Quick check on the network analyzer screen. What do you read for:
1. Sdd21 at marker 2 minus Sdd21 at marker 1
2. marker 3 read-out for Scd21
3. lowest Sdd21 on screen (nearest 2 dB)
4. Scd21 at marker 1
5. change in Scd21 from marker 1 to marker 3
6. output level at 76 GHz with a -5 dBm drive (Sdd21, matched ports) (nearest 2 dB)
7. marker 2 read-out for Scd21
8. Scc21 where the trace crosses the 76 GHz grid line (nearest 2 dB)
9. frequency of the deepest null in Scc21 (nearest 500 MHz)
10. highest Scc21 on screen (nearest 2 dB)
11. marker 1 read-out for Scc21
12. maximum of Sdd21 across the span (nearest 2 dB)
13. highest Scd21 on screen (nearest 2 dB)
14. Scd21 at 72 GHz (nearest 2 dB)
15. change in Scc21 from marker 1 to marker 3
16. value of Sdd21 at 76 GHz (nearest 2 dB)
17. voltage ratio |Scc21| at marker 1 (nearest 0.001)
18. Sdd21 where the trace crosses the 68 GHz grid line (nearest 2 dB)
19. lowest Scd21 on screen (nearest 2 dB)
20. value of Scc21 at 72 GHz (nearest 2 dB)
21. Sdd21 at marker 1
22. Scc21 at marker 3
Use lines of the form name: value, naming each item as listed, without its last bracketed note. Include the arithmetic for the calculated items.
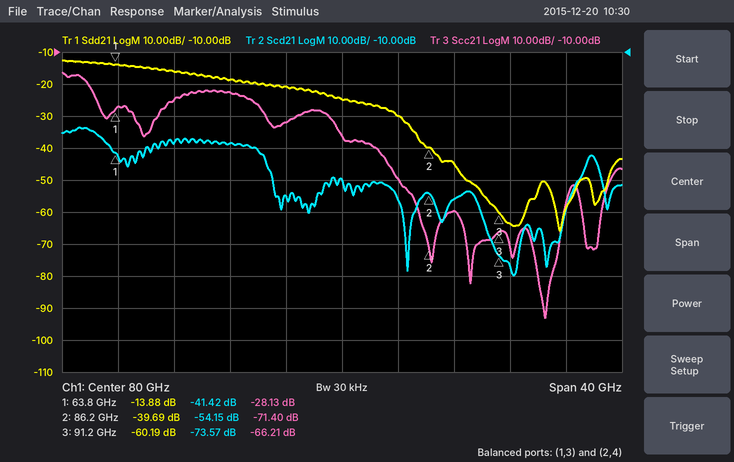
Sdd21 at marker 2 minus Sdd21 at marker 1: -39.69 − (-13.88) = -25.81 dB
marker 3 read-out for Scd21: -73.57 dB
lowest Sdd21 on screen: -66 dB
Scd21 at marker 1: -41.42 dB
change in Scd21 from marker 1 to marker 3: -73.57 − (-41.42) = -32.15 dB
output level at 76 GHz with a -5 dBm drive (Sdd21, matched ports): -5 dBm + (-20 dB) = -26 dBm
marker 2 read-out for Scd21: -54.15 dB
Scc21 where the trace crosses the 76 GHz grid line: -32 dB
frequency of the deepest null in Scc21: 94.5 GHz
highest Scc21 on screen: -16 dB
marker 1 read-out for Scc21: -28.13 dB
maximum of Sdd21 across the span: -12 dB
highest Scd21 on screen: -34 dB
Scd21 at 72 GHz: -38 dB
change in Scc21 from marker 1 to marker 3: -66.21 − (-28.13) = -38.08 dB
value of Sdd21 at 76 GHz: -20 dB
voltage ratio |Scc21| at marker 1: 10^(-28.13/20) ≈ 0.039
Sdd21 where the trace crosses the 68 GHz grid line: -16 dB
lowest Scd21 on screen: -80 dB
value of Scc21 at 72 GHz: -22 dB
Sdd21 at marker 1: -13.88 dB
Scc21 at marker 3: -66.21 dB
